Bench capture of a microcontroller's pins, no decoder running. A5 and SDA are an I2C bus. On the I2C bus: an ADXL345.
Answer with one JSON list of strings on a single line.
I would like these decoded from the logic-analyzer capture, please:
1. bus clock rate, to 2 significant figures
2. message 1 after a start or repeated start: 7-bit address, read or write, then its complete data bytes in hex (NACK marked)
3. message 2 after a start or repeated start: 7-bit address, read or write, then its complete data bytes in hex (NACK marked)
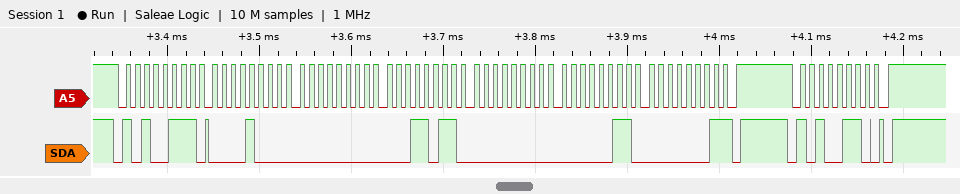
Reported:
["100 kHz", "0x53 read: 08 00 1B 00 03 01 NACK", "0x53 write"]
